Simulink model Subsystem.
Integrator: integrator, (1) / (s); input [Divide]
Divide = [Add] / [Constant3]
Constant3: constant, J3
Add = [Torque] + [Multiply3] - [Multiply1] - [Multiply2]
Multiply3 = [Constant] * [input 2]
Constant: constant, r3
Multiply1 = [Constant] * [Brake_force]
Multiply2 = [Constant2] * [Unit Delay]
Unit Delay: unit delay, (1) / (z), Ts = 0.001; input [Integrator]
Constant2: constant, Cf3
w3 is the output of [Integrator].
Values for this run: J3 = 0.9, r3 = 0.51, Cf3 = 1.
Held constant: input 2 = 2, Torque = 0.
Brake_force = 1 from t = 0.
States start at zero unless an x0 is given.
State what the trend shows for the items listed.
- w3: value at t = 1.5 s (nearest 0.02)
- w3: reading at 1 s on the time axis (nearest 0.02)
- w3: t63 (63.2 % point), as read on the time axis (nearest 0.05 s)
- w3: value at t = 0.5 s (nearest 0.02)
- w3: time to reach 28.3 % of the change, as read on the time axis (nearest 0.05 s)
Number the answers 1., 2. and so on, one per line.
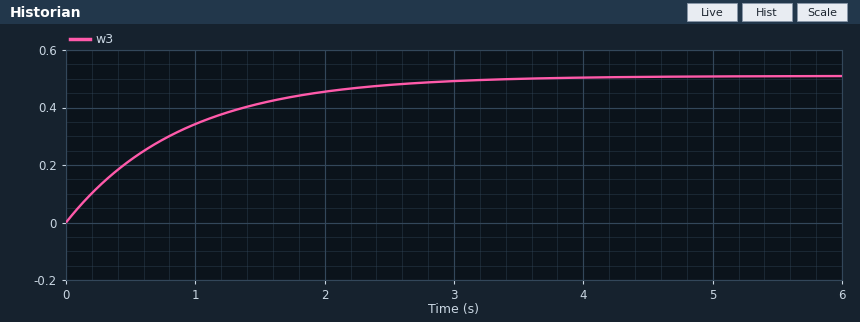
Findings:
1. 0.42
2. 0.34
3. 0.90 s
4. 0.22
5. 0.30 s
